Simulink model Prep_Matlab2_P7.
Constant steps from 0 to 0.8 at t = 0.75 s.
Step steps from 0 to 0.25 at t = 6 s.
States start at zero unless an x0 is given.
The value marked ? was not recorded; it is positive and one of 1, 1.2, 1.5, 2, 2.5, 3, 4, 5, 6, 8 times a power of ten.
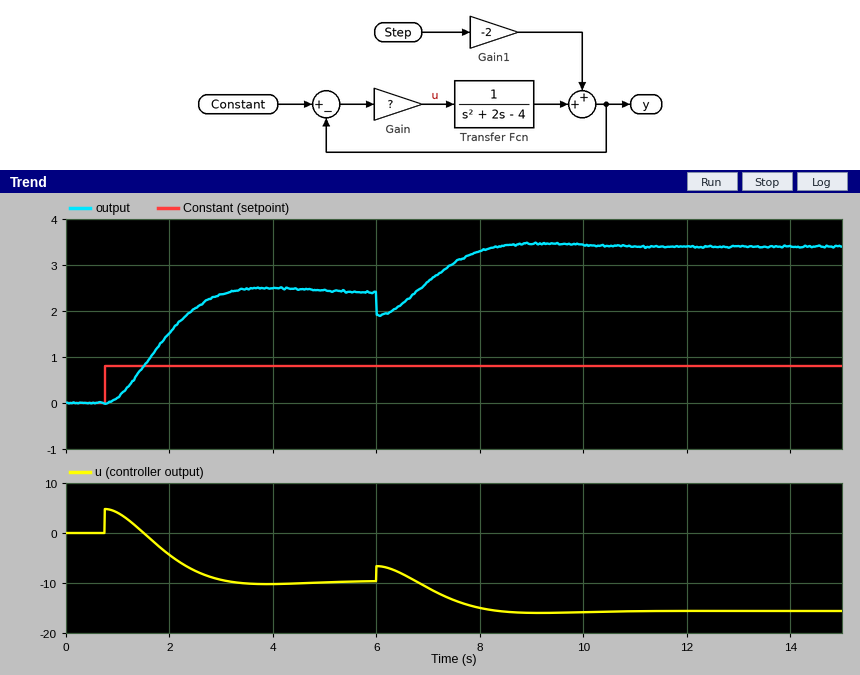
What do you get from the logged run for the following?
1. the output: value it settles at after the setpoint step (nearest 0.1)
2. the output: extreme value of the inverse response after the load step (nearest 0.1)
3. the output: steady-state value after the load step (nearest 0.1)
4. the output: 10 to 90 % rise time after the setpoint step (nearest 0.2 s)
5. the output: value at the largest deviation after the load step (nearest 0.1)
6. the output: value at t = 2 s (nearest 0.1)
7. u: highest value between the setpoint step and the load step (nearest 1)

2.4
1.9
3.4
1.6 s
3.5
1.5
5
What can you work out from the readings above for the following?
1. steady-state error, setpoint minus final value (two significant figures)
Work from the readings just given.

-1.6
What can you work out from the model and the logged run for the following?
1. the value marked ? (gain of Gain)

6
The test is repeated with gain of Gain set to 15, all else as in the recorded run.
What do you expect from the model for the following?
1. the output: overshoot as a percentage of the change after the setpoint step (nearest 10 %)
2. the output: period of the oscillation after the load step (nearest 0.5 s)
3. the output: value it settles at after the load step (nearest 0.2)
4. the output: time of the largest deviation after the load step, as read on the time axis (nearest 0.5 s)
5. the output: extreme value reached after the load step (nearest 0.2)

40 %
2.0 s
1.2
7.0 s
1.6
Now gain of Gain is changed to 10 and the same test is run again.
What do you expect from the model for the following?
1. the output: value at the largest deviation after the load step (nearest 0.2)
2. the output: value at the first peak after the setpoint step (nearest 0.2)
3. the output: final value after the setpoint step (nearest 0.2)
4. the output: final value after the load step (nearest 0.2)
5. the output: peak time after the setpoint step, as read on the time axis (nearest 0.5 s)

1.8
1.6
1.4
1.6
2.0 s
